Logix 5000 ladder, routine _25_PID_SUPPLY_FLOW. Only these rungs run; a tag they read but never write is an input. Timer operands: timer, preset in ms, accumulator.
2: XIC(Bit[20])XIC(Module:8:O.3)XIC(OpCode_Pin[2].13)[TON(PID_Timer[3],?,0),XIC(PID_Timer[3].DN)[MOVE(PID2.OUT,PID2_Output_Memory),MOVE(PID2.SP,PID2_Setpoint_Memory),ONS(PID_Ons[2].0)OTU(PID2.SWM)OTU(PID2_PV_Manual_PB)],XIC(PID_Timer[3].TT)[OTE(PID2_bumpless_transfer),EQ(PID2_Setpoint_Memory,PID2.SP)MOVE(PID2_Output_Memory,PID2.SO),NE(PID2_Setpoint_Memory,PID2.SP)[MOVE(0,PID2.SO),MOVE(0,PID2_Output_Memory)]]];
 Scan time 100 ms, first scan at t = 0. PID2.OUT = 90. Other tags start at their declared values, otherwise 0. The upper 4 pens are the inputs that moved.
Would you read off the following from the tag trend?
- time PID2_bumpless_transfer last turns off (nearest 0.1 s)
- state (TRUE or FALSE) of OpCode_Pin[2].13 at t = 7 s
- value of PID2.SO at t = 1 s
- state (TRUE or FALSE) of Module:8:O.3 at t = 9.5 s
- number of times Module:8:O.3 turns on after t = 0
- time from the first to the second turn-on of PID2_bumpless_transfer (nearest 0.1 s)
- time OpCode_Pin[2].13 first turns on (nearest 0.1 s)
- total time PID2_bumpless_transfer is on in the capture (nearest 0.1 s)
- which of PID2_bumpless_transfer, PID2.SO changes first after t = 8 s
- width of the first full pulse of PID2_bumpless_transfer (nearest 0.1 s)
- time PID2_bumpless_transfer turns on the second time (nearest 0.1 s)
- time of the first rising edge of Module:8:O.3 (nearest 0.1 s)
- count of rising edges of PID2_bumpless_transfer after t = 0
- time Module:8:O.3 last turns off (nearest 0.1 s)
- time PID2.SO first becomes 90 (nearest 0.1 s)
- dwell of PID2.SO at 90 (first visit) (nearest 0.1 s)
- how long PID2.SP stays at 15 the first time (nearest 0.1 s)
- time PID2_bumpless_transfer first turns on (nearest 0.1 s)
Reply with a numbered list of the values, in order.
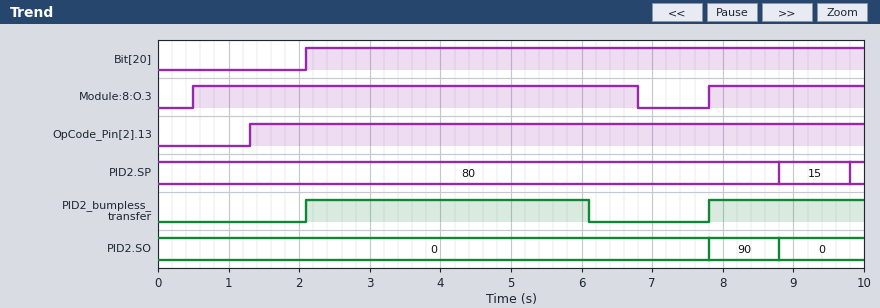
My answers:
1. 6.1 s
2. TRUE
3. 0
4. TRUE
5. 2
6. 5.7 s
7. 1.3 s
8. 6.2 s
9. PID2.SO
10. 4.0 s
11. 7.8 s
12. 0.5 s
13. 2
14. 6.8 s
15. 7.8 s
16. 1.0 s
17. 1.0 s
18. 2.1 s
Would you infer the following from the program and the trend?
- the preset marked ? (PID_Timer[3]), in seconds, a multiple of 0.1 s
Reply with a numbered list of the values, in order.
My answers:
1. 4.0 s
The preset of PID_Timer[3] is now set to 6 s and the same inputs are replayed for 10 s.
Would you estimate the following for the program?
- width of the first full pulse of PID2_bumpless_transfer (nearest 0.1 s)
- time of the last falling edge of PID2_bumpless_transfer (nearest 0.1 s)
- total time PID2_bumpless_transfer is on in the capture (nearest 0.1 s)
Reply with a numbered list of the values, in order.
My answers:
1. 4.7 s
2. 6.8 s
3. 6.9 s
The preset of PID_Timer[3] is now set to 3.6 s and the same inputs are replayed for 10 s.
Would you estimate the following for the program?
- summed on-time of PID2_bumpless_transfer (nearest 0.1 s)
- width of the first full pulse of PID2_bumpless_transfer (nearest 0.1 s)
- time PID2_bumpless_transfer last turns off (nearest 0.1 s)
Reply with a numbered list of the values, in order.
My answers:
1. 5.8 s
2. 3.6 s
3. 5.7 s
